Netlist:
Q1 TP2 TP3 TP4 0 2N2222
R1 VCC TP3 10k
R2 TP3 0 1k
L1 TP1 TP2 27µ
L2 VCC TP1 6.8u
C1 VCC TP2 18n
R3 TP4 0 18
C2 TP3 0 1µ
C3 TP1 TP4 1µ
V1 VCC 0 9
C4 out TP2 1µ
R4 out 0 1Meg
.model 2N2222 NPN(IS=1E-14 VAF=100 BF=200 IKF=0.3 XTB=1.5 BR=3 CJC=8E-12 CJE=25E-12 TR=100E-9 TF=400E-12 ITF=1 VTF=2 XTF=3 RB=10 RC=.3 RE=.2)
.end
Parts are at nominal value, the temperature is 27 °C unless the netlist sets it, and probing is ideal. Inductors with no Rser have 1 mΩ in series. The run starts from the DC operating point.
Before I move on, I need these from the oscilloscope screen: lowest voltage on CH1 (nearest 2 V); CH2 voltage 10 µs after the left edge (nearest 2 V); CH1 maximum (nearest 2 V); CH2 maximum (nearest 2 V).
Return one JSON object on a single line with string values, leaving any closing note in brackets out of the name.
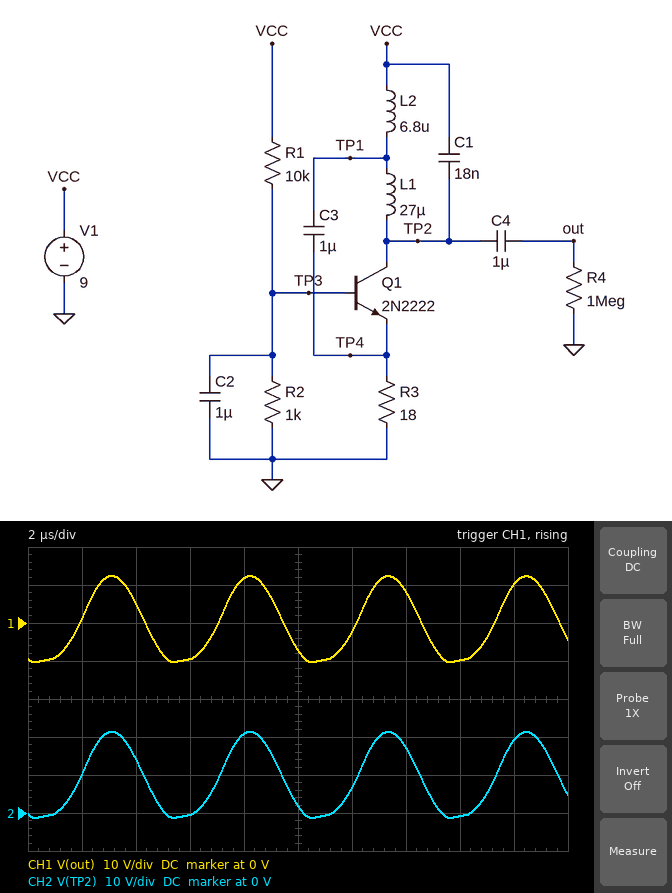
{"lowest voltage on CH1": "-10 V", "CH2 voltage 10 µs after the left edge": "2 V", "CH1 maximum": "12 V", "CH2 maximum": "22 V"}
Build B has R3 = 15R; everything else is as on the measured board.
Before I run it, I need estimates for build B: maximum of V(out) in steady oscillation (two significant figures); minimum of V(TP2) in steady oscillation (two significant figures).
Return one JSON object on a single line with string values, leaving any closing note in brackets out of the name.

{"maximum of V(out) in steady oscillation": "13 V", "minimum of V(TP2) in steady oscillation": "-1.2 V"}
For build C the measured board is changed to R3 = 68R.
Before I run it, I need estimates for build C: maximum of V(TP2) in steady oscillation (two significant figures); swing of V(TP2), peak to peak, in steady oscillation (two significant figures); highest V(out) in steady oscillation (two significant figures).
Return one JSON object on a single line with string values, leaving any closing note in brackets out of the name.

{"maximum of V(TP2) in steady oscillation": "20 V", "swing of V(TP2), peak to peak, in steady oscillation": "21 V", "highest V(out) in steady oscillation": "11 V"}
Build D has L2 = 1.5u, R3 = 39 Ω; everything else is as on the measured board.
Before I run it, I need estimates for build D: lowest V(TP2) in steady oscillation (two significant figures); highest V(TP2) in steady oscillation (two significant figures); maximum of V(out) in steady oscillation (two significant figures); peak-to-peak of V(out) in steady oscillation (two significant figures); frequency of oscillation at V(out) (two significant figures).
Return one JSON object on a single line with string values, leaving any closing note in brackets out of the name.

{"lowest V(TP2) in steady oscillation": "-660 mV", "highest V(TP2) in steady oscillation": "19 V", "maximum of V(out) in steady oscillation": "10 V", "peak-to-peak of V(out) in steady oscillation": "20 V", "frequency of oscillation at V(out)": "220 kHz"}
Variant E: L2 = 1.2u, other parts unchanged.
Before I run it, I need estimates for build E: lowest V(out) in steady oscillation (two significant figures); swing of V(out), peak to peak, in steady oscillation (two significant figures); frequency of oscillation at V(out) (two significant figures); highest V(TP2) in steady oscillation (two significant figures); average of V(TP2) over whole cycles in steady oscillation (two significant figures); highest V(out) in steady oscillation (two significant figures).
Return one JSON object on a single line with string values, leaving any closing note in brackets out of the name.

{"lowest V(out) in steady oscillation": "-9.7 V", "swing of V(out), peak to peak, in steady oscillation": "20 V", "frequency of oscillation at V(out)": "220 kHz", "highest V(TP2) in steady oscillation": "19 V", "average of V(TP2) over whole cycles in steady oscillation": "9.0 V", "highest V(out) in steady oscillation": "10 V"}
